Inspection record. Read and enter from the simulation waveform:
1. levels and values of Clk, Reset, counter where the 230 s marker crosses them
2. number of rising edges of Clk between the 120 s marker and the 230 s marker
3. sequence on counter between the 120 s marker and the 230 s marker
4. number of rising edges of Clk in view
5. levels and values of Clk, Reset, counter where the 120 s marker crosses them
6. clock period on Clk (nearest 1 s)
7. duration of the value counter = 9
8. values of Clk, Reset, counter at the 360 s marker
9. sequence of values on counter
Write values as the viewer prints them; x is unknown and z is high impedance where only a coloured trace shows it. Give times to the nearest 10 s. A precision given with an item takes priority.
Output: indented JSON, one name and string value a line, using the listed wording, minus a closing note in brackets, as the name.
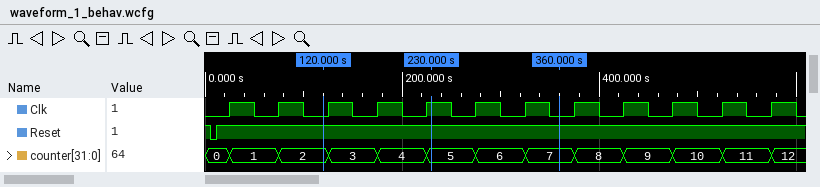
{
  "levels and values of Clk, Reset, counter where the 230 s marker crosses them": "Clk=1, Reset=1, counter=5",
  "number of rising edges of Clk between the 120 s marker and the 230 s marker": "3",
  "sequence on counter between the 120 s marker and the 230 s marker": "2, 3, 4, 5",
  "number of rising edges of Clk in view": "12",
  "levels and values of Clk, Reset, counter where the 120 s marker crosses them": "Clk=0, Reset=1, counter=2",
  "clock period on Clk": "50 s",
  "duration of the value counter = 9": "50 s",
  "values of Clk, Reset, counter at the 360 s marker": "Clk=0, Reset=1, counter=7",
  "sequence of values on counter": "0, 1, 2, 3, 4, 5, 6, 7, 8, 9, 10, 11, 12"
}
